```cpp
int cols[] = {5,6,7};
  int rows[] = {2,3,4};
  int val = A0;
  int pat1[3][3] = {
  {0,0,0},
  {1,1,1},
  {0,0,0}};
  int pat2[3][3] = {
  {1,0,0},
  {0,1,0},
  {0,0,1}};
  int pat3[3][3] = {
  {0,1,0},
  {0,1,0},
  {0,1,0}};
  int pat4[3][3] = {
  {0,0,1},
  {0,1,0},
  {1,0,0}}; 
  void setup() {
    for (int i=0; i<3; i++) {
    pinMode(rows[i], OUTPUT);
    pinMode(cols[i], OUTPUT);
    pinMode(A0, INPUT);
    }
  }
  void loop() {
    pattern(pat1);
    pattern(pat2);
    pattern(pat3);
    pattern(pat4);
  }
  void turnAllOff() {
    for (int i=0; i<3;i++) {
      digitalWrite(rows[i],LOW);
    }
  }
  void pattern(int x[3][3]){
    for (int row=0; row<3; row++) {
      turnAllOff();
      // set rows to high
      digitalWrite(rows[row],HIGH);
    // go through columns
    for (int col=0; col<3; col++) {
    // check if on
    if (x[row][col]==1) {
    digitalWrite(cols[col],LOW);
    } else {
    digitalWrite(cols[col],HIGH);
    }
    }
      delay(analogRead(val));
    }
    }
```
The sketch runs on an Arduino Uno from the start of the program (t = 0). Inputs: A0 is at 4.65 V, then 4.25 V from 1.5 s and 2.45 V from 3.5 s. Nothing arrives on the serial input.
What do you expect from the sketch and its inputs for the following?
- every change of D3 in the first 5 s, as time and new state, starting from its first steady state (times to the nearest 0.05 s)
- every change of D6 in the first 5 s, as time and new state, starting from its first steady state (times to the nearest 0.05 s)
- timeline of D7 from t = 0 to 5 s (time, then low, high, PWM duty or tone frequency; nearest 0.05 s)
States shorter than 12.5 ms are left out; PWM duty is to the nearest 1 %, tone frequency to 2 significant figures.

0 s low; 0.95 s high; 1.9 s low; 3.65 s high; 4.15 s low
0 s high; 0.95 s low; 1.9 s high; 3.65 s low; 4.15 s high; 4.65 s low
0 s high; 0.95 s low; 1.9 s high; 4.15 s low; 4.65 s high
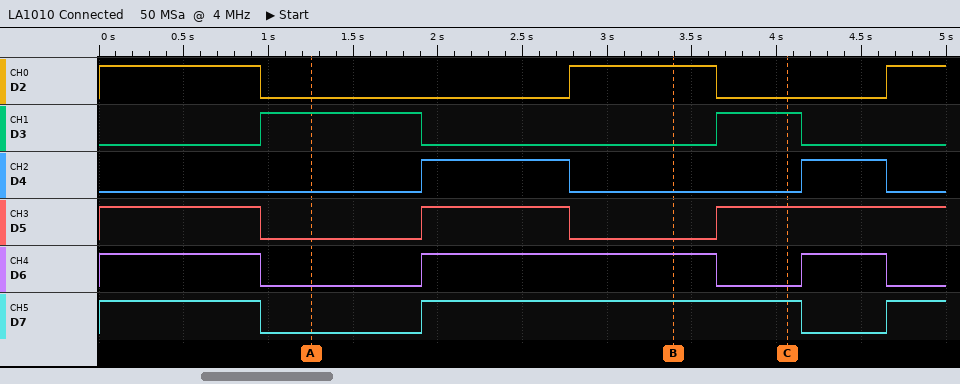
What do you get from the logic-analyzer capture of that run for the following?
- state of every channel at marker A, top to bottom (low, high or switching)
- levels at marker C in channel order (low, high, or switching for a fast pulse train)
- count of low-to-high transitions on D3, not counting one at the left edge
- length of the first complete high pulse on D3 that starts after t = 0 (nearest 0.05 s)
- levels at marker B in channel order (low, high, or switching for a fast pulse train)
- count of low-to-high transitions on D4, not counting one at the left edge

D2 low, D3 high, D4 low, D5 low, D6 low, D7 low
D2 low, D3 high, D4 low, D5 high, D6 low, D7 high
2
0.95 s
D2 high, D3 low, D4 low, D5 low, D6 high, D7 high
2
